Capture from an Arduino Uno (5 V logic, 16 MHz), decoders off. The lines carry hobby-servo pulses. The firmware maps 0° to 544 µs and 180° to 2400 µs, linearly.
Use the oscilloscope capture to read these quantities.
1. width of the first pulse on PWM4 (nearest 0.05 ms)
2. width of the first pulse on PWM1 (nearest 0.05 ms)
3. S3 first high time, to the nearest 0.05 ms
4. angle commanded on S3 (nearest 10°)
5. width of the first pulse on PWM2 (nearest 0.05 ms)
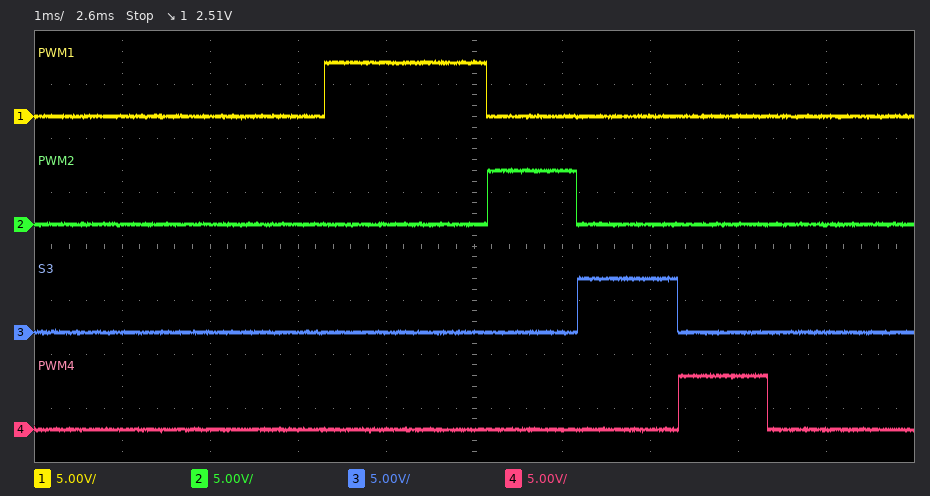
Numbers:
1.00 ms
1.85 ms
1.15 ms
60°
1.00 ms
